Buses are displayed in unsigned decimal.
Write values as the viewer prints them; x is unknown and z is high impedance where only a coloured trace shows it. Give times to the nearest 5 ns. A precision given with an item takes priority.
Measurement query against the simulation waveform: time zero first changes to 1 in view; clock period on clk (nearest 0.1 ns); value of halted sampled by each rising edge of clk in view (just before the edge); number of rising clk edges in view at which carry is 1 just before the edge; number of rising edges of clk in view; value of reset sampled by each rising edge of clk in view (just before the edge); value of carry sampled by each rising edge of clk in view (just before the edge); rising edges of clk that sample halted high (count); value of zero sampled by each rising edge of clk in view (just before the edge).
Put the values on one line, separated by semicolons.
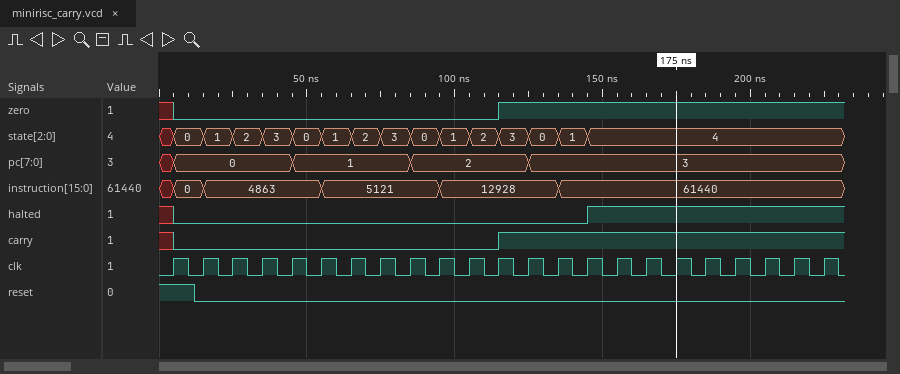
115 ns; 10 ns; x 0 0 0 0 0 0 0 0 0 0 0 0 0 0 1 1 1 1 1 1 1 1; 11; 23; 1 0 0 0 0 0 0 0 0 0 0 0 0 0 0 0 0 0 0 0 0 0 0; x 0 0 0 0 0 0 0 0 0 0 0 1 1 1 1 1 1 1 1 1 1 1; 8; x 0 0 0 0 0 0 0 0 0 0 0 1 1 1 1 1 1 1 1 1 1 1
